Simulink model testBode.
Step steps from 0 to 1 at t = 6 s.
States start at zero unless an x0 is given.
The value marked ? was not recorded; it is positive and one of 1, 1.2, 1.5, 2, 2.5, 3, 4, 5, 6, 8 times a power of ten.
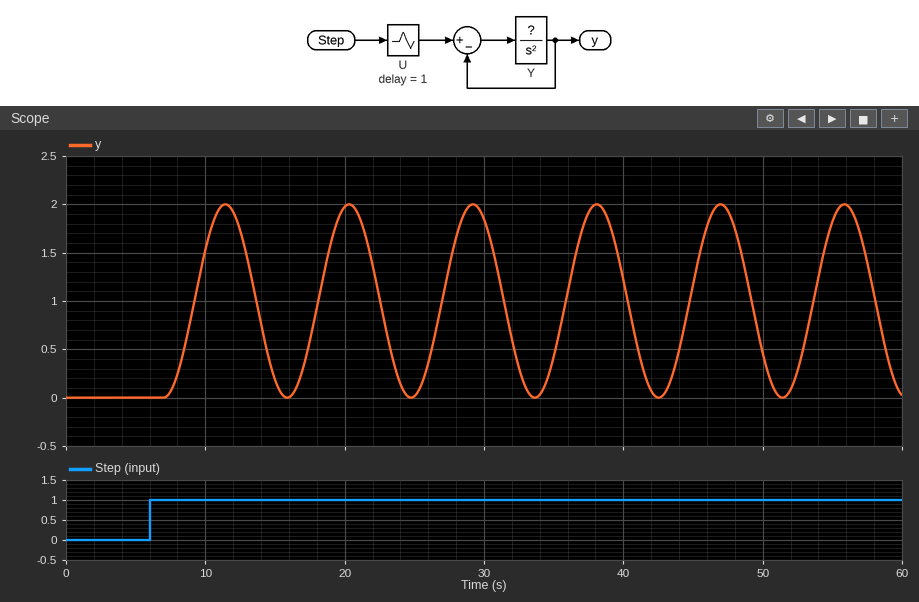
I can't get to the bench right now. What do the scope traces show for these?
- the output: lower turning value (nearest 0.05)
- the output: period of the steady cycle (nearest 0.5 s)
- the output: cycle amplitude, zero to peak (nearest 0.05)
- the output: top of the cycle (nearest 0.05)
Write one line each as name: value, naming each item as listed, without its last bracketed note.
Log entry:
the output: lower turning value: 0.00
the output: period of the steady cycle: 9.0 s
the output: cycle amplitude, zero to peak: 1.00
the output: top of the cycle: 2.00
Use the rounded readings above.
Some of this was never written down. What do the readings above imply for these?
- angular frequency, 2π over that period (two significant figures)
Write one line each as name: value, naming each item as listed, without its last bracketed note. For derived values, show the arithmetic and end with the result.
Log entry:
angular frequency, 2π over that period: 2π / 9 = 0.70 rad/s
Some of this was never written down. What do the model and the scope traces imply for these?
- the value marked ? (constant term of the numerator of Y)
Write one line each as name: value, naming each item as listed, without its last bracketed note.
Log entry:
the value marked ?: 0.5
